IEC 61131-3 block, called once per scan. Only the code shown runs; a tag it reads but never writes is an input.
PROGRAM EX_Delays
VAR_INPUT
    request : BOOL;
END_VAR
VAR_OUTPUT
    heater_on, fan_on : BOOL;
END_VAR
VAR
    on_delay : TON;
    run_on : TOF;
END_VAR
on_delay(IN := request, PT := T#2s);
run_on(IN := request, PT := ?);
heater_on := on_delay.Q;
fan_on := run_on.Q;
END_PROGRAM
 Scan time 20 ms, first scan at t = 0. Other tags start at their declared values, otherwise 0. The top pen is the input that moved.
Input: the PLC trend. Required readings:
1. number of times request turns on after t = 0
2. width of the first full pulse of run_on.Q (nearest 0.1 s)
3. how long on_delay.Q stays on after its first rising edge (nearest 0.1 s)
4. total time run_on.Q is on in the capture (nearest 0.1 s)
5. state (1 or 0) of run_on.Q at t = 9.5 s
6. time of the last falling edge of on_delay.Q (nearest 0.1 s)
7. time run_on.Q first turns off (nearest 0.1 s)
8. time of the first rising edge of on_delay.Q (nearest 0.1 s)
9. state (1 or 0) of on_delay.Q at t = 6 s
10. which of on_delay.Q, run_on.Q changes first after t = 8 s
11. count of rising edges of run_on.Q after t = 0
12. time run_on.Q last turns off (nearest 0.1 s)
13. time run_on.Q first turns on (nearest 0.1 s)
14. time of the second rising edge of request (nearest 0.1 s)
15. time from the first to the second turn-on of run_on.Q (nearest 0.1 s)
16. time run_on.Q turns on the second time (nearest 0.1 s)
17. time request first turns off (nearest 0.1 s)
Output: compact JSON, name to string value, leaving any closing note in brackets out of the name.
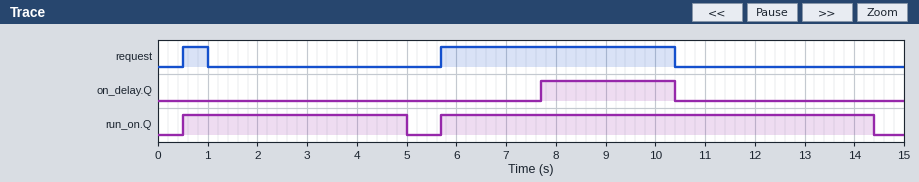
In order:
{"number of times request turns on after t = 0": "2", "width of the first full pulse of run_on.Q": "4.5 s", "how long on_delay.Q stays on after its first rising edge": "2.7 s", "total time run_on.Q is on in the capture": "13.2 s", "state (1 or 0) of run_on.Q at t = 9.5 s": "1", "time of the last falling edge of on_delay.Q": "10.4 s", "time run_on.Q first turns off": "5.0 s", "time of the first rising edge of on_delay.Q": "7.7 s", "state (1 or 0) of on_delay.Q at t = 6 s": "0", "which of on_delay.Q, run_on.Q changes first after t = 8 s": "on_delay.Q", "count of rising edges of run_on.Q after t = 0": "2", "time run_on.Q last turns off": "14.4 s", "time run_on.Q first turns on": "0.5 s", "time of the second rising edge of request": "5.7 s", "time from the first to the second turn-on of run_on.Q": "5.2 s", "time run_on.Q turns on the second time": "5.7 s", "time request first turns off": "1.0 s"}
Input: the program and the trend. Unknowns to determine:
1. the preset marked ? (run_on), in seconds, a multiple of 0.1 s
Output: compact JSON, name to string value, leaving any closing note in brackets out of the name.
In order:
{"the preset marked ? (run_on), in seconds, a multiple of 0.1 s": "4.0 s"}
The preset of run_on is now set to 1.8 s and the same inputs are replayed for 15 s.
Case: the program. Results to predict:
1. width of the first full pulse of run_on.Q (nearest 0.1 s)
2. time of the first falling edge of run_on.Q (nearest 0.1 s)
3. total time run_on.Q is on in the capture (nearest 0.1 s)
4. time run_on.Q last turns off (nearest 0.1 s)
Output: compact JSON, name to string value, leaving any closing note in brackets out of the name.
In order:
{"width of the first full pulse of run_on.Q": "2.3 s", "time of the first falling edge of run_on.Q": "2.8 s", "total time run_on.Q is on in the capture": "8.8 s", "time run_on.Q last turns off": "12.2 s"}
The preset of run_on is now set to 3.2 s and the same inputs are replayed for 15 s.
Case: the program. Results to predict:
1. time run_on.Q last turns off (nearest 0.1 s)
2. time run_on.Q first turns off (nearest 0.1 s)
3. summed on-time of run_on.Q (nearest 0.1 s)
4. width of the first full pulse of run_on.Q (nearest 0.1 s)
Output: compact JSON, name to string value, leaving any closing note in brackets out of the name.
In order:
{"time run_on.Q last turns off": "13.6 s", "time run_on.Q first turns off": "4.2 s", "summed on-time of run_on.Q": "11.6 s", "width of the first full pulse of run_on.Q": "3.7 s"}
